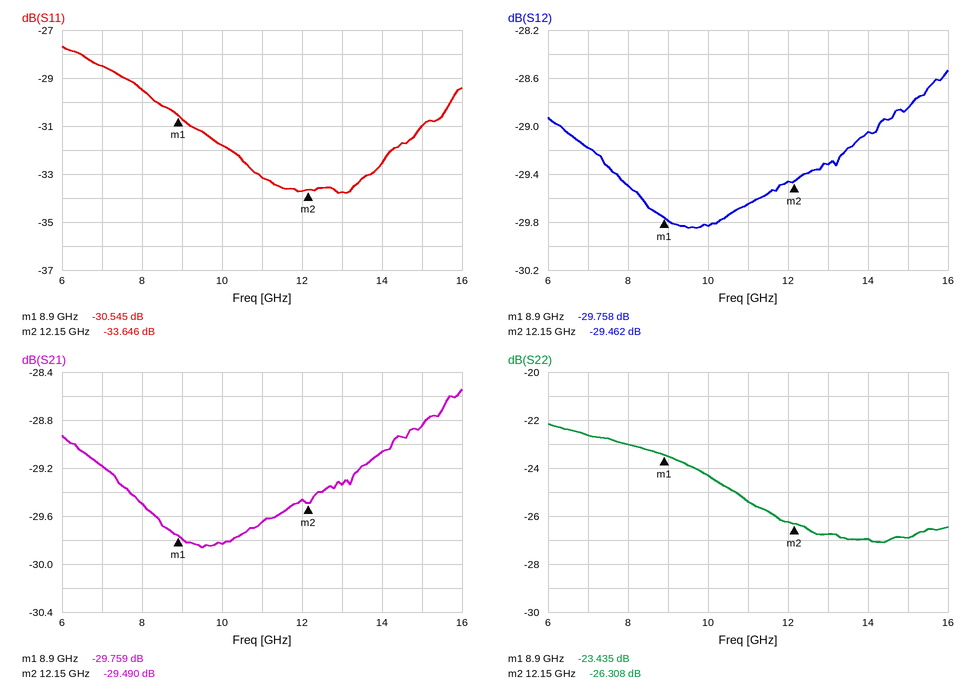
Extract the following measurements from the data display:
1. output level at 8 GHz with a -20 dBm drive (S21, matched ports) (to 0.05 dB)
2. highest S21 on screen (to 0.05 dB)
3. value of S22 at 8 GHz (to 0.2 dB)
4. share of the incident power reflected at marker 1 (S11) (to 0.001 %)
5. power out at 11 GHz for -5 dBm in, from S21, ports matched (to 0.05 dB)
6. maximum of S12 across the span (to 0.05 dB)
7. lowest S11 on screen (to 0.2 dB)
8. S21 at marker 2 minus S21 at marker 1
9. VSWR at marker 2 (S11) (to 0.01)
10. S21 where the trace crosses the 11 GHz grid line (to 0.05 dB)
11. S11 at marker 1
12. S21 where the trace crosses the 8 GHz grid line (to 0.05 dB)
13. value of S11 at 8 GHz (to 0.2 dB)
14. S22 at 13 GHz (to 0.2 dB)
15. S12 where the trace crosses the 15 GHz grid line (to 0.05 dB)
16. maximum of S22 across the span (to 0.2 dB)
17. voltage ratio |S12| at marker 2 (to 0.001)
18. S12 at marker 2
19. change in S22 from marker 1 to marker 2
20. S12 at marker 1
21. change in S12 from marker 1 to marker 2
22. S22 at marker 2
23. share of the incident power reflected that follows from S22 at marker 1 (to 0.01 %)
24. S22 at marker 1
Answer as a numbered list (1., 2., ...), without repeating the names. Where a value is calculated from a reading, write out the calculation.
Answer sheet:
1. -20 dBm + (-29.50 dB) = -49.50 dBm
2. -28.55 dB
3. -23.0 dB
4. 10^(-30.545/10) ≈ 0.088 %
5. -5 dBm + (-29.65 dB) = -34.65 dBm
6. -28.55 dB
7. -33.8 dB
8. -29.49 − (-29.759) = 0.269 dB
9. (1 + 0.0208)/(1 − 0.0208) ≈ 1.04
10. -29.65 dB
11. -30.545 dB
12. -29.50 dB
13. -29.4 dB
14. -26.8 dB
15. -28.85 dB
16. -22.2 dB
17. 10^(-29.462/20) ≈ 0.034
18. -29.462 dB
19. -26.308 − (-23.435) = -2.873 dB
20. -29.758 dB
21. -29.462 − (-29.758) = 0.296 dB
22. -26.308 dB
23. 10^(-23.435/10) ≈ 0.45 %
24. -23.435 dB
